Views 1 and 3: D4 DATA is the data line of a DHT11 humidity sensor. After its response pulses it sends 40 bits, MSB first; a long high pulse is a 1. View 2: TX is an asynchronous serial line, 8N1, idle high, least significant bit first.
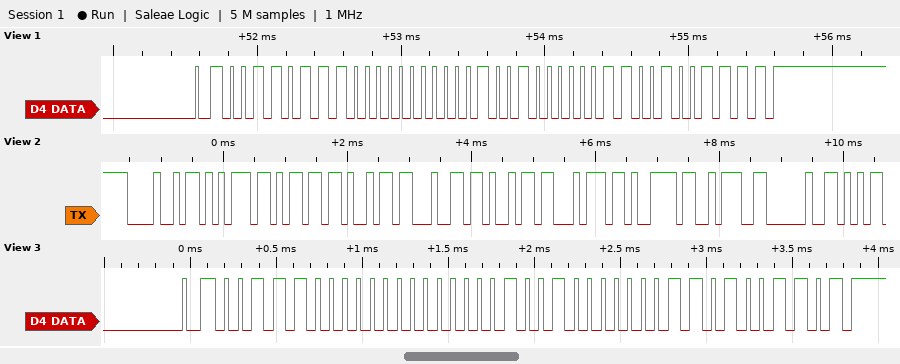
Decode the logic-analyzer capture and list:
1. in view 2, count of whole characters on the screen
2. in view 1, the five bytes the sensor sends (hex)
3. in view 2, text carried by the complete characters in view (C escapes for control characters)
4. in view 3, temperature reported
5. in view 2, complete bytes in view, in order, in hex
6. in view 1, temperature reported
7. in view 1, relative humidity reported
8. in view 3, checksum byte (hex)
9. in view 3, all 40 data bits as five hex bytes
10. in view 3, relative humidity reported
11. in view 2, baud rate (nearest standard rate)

10
37 00 12 06 4F
"Humidity: "
18.3 °C
48 75 6D 69 64 69 74 79 3A 20
18.6 °C
55 %
0x4D
38 00 12 03 4D
56 %
9600 baud
